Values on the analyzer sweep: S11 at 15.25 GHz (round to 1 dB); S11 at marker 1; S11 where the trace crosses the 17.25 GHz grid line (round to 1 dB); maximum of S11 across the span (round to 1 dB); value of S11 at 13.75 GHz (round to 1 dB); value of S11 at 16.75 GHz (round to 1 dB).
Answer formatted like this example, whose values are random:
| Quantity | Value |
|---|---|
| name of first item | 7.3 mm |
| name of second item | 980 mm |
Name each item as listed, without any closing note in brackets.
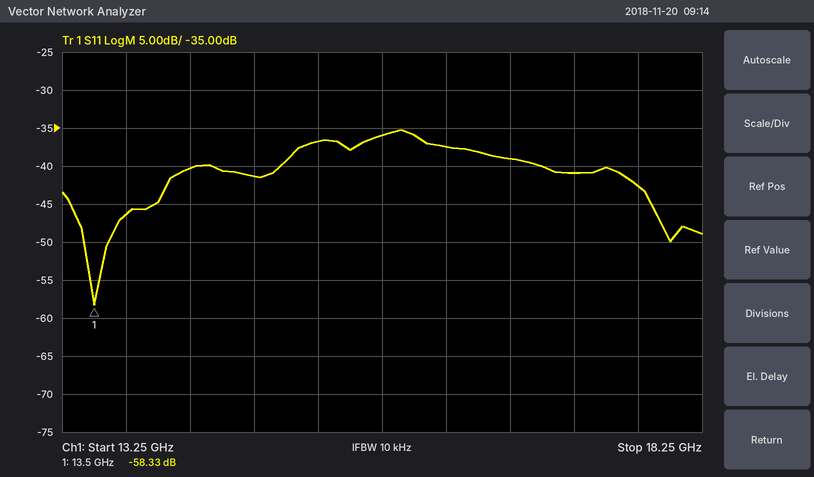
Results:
| Quantity | Value |
|---|---|
| S11 at 15.25 GHz | -37 dB |
| S11 at marker 1 | -58.33 dB |
| S11 where the trace crosses the 17.25 GHz grid line | -41 dB |
| maximum of S11 across the span | -35 dB |
| value of S11 at 13.75 GHz | -46 dB |
| value of S11 at 16.75 GHz | -39 dB |
